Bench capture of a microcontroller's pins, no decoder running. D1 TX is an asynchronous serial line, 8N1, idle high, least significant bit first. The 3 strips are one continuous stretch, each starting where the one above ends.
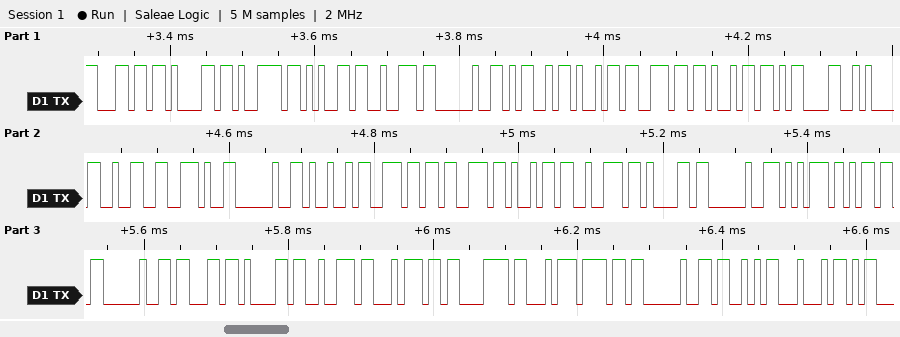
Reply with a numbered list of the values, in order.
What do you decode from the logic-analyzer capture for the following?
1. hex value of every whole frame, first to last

1. 6C 61 79 65 72 20 4D 69 6E 69 0D 0A 32 2E 20 49 6E 73 69 72 61 20 75 6D 20 63 61 72 74 C3 A3 6F 20 53 44
